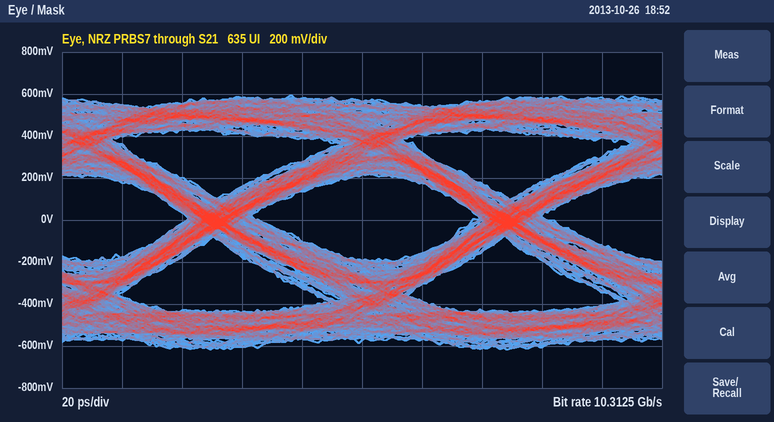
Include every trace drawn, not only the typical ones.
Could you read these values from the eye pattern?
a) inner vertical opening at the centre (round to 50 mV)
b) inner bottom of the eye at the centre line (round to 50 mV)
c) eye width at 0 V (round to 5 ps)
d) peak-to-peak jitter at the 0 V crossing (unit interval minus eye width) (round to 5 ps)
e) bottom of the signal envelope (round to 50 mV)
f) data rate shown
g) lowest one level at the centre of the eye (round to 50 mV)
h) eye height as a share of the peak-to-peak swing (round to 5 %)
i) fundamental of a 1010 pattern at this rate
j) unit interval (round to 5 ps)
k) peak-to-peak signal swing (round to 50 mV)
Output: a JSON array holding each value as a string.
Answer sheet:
["400 mV", "-200 mV", "70 ps", "25 ps", "-600 mV", "10.3125 Gb/s", "200 mV", "35 %", "5.15625 GHz", "95 ps", "1.20 V"]
